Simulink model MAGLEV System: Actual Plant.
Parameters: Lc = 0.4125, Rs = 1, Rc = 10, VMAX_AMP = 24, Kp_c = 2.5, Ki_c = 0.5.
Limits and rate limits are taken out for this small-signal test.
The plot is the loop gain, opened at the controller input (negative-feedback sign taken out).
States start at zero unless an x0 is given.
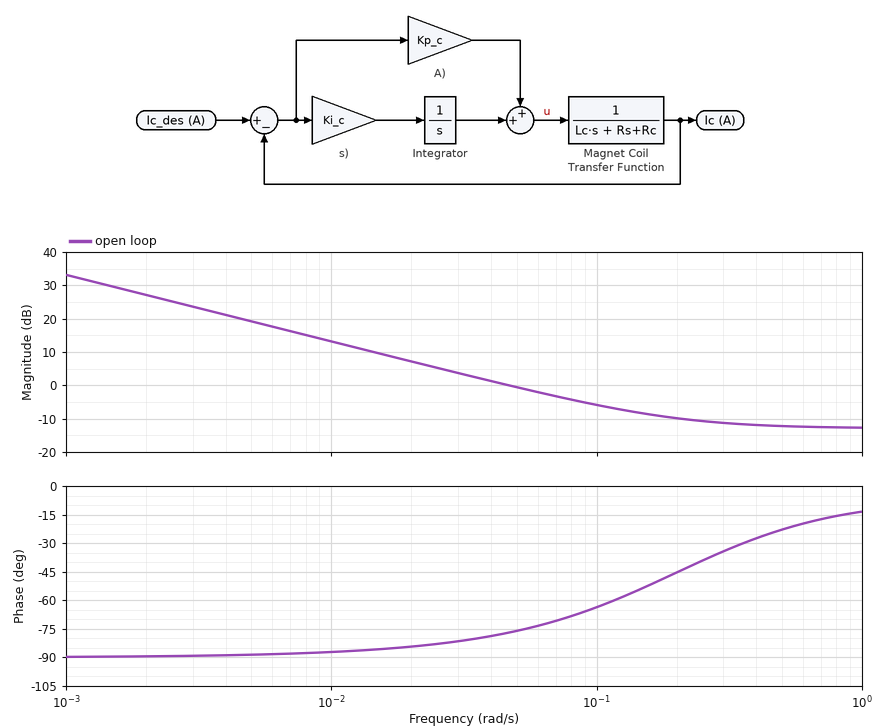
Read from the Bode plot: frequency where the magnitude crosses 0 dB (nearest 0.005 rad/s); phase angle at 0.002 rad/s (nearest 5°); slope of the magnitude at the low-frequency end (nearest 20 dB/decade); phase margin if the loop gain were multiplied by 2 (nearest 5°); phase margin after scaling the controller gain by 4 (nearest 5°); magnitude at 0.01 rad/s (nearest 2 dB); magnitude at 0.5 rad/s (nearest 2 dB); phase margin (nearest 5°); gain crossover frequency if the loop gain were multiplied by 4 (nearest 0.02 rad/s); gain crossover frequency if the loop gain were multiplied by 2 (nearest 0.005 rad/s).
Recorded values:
0.045 rad/s
-90°
-20 dB/decade
115°
155°
14 dB
-12 dB
105°
0.44 rad/s
0.100 rad/s
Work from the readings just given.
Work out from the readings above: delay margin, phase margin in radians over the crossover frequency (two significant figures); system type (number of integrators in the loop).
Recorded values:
41 s
1
